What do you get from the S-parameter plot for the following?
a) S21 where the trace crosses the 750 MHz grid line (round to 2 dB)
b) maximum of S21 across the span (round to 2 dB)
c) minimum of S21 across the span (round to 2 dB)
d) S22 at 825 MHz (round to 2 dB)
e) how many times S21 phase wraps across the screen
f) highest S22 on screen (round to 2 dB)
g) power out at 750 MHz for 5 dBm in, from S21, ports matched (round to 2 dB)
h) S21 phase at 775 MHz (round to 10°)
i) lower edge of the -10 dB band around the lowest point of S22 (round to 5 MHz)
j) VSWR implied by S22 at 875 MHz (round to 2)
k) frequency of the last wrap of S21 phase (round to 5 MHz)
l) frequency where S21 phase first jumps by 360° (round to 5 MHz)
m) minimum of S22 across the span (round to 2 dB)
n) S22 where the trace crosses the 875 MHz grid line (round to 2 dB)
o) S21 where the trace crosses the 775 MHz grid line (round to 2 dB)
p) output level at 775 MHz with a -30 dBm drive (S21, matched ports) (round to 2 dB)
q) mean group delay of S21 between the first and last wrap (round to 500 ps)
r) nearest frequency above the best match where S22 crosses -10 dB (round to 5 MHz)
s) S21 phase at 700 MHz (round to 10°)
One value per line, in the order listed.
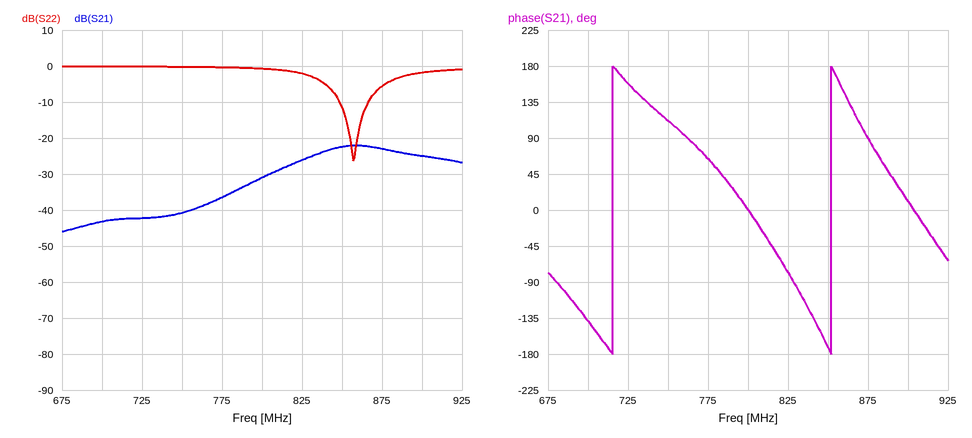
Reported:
-40 dB
-22 dB
-46 dB
-2 dB
2
0 dB
-36 dBm
60°
850 MHz
4
850 MHz
715 MHz
-26 dB
-6 dB
-36 dB
-66 dBm
7.5 ns
865 MHz
-140°
